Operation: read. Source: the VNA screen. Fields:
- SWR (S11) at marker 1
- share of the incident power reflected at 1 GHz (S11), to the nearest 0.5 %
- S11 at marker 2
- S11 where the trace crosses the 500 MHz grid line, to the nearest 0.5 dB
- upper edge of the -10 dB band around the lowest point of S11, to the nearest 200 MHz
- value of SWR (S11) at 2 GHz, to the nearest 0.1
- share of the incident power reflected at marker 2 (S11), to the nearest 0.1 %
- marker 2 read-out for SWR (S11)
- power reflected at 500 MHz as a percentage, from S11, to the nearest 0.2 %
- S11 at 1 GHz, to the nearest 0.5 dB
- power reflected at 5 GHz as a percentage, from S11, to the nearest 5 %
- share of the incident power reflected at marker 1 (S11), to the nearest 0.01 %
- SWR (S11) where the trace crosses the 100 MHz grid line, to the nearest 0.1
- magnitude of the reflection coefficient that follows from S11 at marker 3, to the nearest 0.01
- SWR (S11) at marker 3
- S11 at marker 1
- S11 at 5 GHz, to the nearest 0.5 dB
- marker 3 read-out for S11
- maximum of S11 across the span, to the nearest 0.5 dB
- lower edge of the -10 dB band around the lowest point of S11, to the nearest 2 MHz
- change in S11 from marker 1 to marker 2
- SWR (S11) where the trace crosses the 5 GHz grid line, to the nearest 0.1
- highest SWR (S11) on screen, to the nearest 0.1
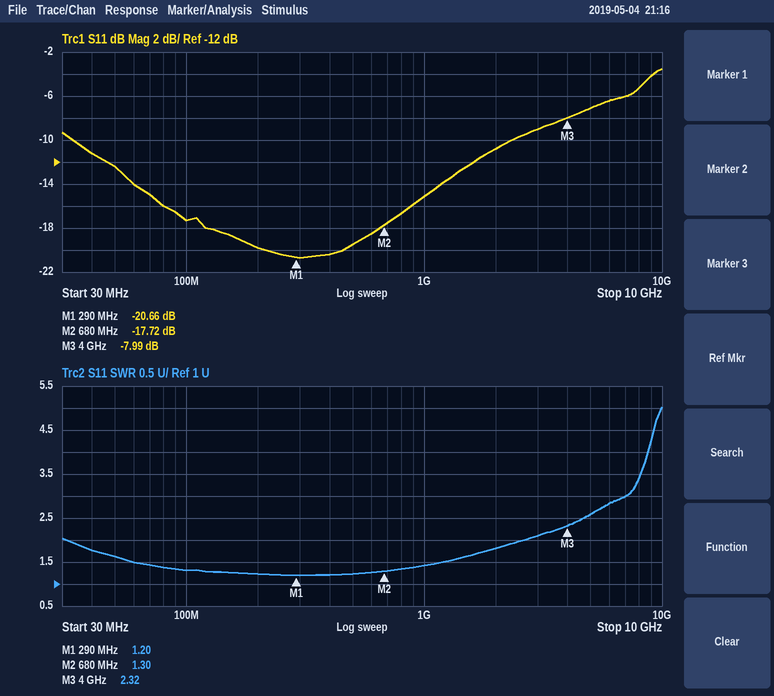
1.20
3.0 %
-17.72 dB
-19.5 dB
2.4 GHz
1.8
1.7 %
1.30
1.2 %
-15.0 dB
20 %
0.86 %
1.3
0.40
2.32
-20.66 dB
-7.0 dB
-7.99 dB
-3.5 dB
34 MHz
2.94 dB
2.6
5.0
